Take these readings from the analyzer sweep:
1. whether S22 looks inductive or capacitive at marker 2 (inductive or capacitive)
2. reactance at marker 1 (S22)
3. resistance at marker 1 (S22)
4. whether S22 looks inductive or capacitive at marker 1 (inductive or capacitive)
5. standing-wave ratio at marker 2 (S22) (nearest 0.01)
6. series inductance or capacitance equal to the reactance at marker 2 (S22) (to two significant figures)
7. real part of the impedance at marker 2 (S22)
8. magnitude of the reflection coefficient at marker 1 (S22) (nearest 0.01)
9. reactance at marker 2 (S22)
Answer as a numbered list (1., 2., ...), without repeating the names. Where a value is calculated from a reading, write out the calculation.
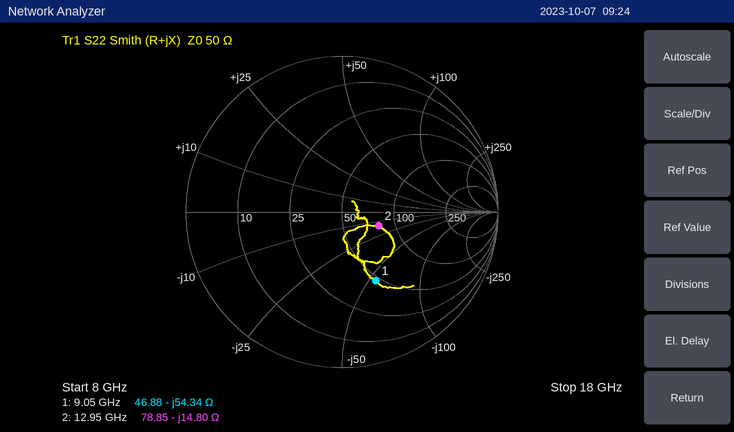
1. capacitive
2. -54.34 Ω
3. 46.88 Ω
4. capacitive
5. 1.67
6. C = 1/(2π × 12.95 GHz × 14.8 Ω) ≈ 830 fF
7. 78.85 Ω
8. 0.49
9. -14.80 Ω
